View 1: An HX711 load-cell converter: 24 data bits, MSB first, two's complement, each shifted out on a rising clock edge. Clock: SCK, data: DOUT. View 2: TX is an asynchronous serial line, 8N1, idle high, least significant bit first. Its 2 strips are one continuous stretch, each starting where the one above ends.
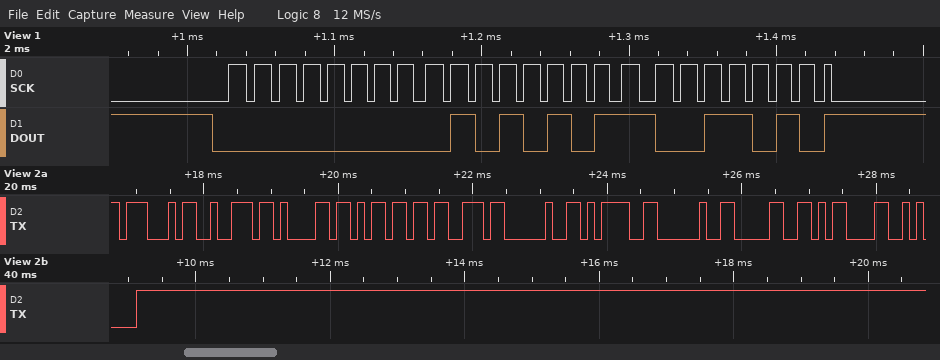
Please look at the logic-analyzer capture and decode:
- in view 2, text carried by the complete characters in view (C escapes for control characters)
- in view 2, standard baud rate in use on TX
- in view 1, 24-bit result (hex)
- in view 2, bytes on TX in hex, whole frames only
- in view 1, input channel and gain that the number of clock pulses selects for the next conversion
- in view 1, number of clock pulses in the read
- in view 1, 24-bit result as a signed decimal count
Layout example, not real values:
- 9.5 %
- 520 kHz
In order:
- "Grams = 0\r\n"
- 9600 baud
- 0x00559A
- 47 72 61 6D 73 20 3D 20 30 0D 0A
- channel A, gain 128
- 25
- 21914
